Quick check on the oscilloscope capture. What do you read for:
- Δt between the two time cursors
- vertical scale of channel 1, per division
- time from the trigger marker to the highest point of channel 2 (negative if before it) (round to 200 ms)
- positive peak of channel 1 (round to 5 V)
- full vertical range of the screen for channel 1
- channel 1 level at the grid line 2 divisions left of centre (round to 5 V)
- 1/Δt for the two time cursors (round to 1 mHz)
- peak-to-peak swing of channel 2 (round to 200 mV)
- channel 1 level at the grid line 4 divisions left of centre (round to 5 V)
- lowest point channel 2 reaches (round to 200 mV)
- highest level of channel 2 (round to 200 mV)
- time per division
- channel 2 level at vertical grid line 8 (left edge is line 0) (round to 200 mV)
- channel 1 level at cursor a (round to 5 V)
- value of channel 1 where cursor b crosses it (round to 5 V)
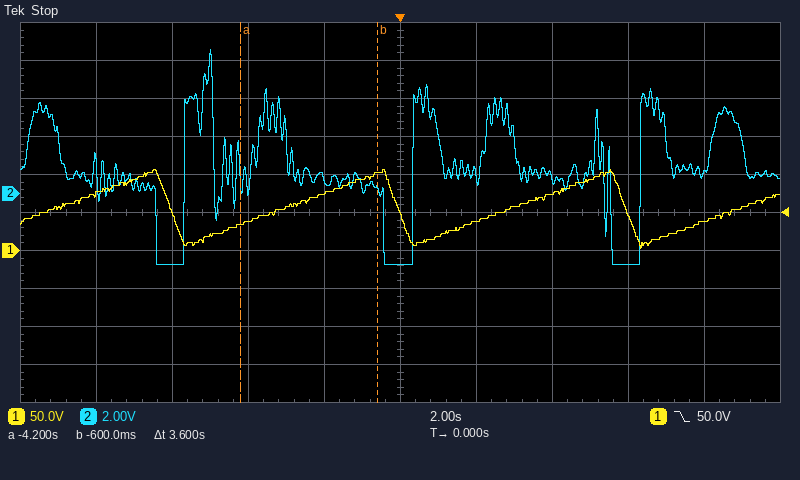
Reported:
3.6 s
50 V
-5.0 s
105 V
500 V
40 V
278 mHz
11.4 V
75 V
-3.8 V
7.6 V
2 s
-3.8 V
35 V
100 V
